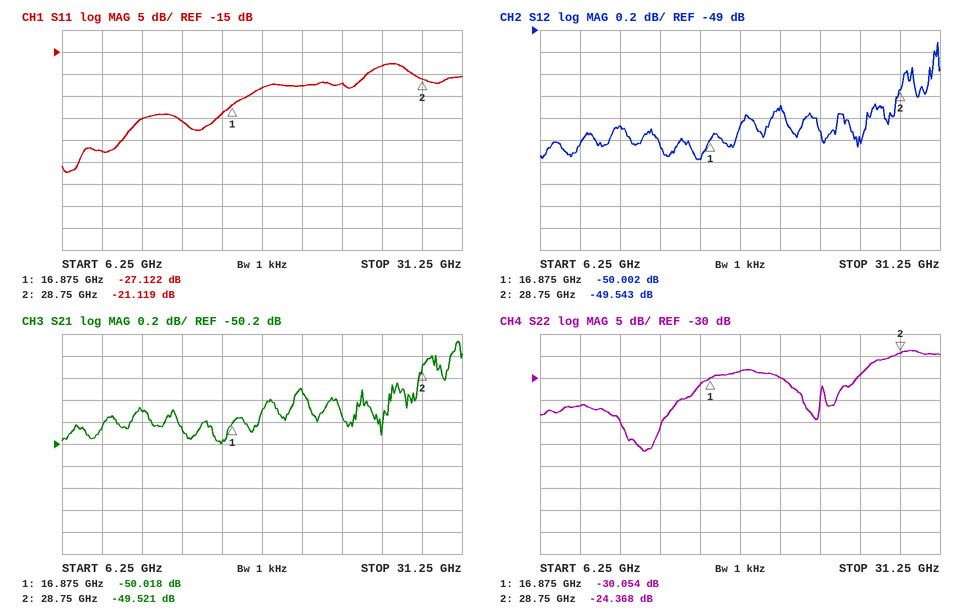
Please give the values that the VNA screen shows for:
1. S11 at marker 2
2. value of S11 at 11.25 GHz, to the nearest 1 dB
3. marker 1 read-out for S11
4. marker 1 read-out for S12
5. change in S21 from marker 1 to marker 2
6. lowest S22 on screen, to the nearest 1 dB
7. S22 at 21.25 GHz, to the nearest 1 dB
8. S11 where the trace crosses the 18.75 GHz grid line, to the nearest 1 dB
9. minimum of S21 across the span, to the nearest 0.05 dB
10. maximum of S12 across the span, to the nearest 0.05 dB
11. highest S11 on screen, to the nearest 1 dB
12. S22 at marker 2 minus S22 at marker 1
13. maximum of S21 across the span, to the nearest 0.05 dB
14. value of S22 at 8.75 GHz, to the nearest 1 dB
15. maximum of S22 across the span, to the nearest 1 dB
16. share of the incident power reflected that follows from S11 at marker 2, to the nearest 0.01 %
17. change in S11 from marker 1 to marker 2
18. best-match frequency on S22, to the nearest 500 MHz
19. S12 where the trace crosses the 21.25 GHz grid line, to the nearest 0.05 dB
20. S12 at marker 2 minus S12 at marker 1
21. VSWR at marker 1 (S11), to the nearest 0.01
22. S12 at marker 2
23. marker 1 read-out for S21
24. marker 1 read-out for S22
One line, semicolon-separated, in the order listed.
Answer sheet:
-21.119 dB; -30 dB; -27.122 dB; -50.002 dB; 0.497 dB; -47 dB; -30 dB; -23 dB; -50.20 dB; -49.10 dB; -18 dB; 5.686 dB; -49.25 dB; -36 dB; -24 dB; 0.77 %; 6.003 dB; 13.0 GHz; -49.70 dB; 0.459 dB; 1.09; -49.543 dB; -50.018 dB; -30.054 dB
